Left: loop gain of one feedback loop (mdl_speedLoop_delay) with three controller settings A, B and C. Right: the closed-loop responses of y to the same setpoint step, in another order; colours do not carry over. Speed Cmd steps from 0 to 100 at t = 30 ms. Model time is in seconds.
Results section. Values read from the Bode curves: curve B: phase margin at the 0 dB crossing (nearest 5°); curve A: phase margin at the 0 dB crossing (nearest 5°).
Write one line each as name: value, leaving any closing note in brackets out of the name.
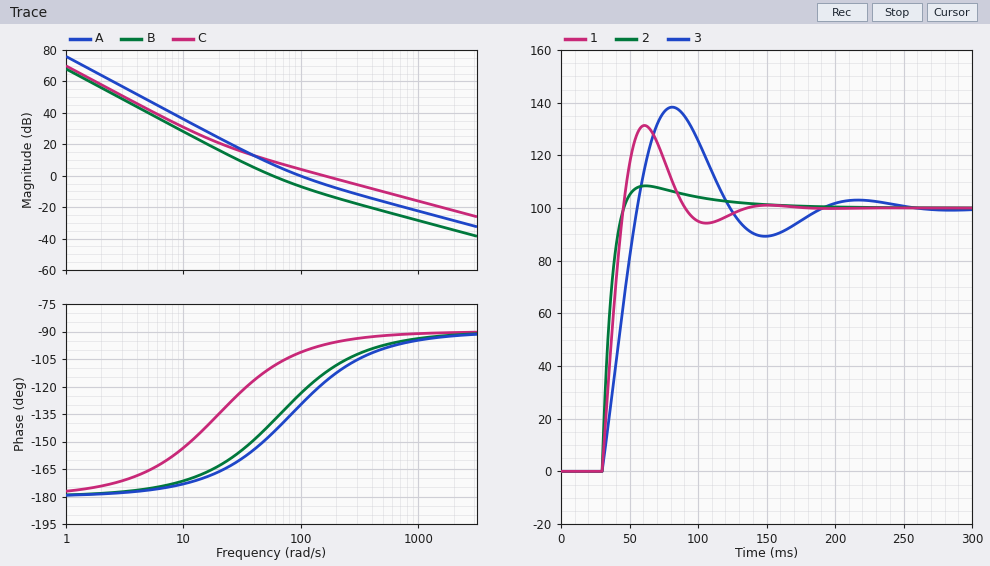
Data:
curve B: phase margin at the 0 dB crossing: 40°
curve A: phase margin at the 0 dB crossing: 50°
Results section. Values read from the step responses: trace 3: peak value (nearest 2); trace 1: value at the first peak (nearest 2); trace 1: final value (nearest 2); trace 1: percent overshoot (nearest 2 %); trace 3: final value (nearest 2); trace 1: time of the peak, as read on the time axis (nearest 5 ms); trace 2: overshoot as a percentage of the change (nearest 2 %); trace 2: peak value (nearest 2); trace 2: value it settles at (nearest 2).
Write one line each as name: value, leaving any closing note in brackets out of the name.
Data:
trace 3: peak value: 138
trace 1: value at the first peak: 132
trace 1: final value: 100
trace 1: percent overshoot: 32 %
trace 3: final value: 100
trace 1: time of the peak, as read on the time axis: 60 ms
trace 2: overshoot as a percentage of the change: 8 %
trace 2: peak value: 108
trace 2: value it settles at: 100
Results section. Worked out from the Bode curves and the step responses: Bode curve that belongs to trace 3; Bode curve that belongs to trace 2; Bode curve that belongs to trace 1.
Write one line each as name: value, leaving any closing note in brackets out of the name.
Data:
Bode curve that belongs to trace 3: B
Bode curve that belongs to trace 2: C
Bode curve that belongs to trace 1: A
